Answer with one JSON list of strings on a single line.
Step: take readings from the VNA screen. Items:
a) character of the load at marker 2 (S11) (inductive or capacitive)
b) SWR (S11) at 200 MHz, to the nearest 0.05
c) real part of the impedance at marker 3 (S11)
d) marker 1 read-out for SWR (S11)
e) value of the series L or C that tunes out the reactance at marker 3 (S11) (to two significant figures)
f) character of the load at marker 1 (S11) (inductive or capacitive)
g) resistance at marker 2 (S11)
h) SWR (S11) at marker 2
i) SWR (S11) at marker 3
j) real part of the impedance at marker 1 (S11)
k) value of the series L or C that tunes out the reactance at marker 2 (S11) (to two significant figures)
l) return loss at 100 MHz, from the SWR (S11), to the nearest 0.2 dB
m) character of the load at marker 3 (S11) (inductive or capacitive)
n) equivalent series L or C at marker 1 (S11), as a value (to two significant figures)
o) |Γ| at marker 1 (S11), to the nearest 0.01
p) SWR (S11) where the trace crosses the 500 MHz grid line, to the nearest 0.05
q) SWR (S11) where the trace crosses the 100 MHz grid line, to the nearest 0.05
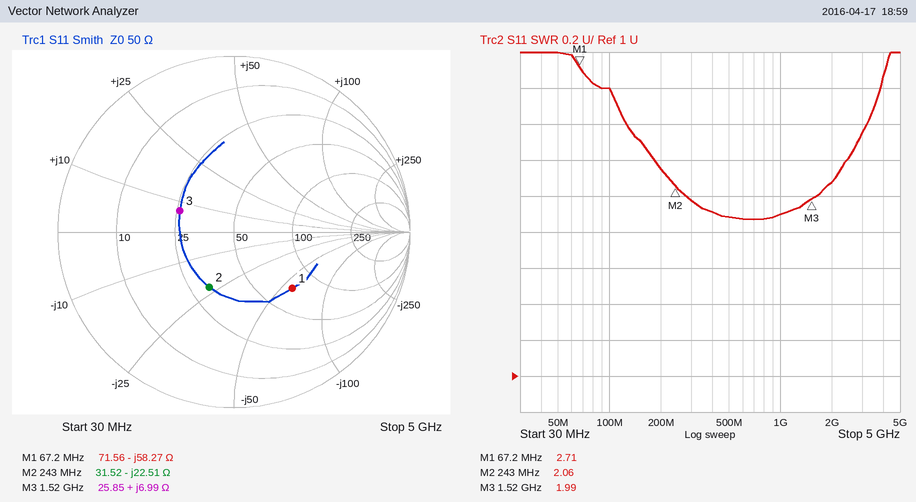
["capacitive", "2.15", "25.85 Ω", "2.71", "15 pF", "capacitive", "31.52 Ω", "2.06", "1.99", "71.56 Ω", "15 nH", "7.0 dB", "inductive", "41 pF", "0.46", "1.90", "2.60"]
